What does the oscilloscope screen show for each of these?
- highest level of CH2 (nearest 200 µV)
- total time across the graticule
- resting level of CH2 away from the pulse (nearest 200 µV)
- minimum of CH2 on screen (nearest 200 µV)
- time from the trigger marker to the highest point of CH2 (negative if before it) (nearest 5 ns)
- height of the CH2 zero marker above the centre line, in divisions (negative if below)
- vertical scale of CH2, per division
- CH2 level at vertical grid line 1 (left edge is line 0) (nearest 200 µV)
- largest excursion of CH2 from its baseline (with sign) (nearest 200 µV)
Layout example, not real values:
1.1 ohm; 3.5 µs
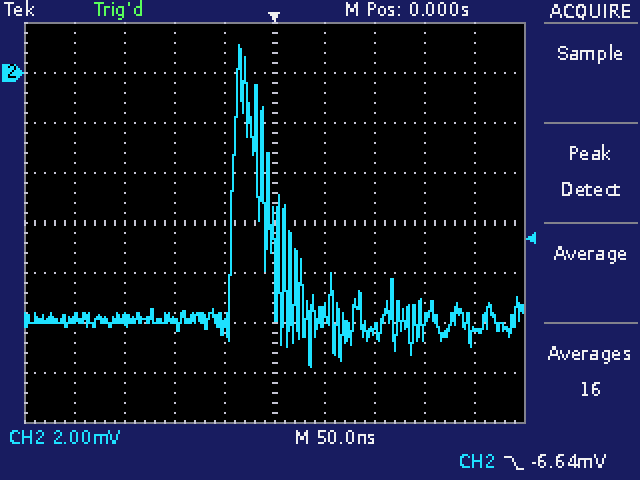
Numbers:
1.2 mV; 500 ns; -9.8 mV; -11.8 mV; -35 ns; +3.0 div; 2 mV; -9.8 mV; +11.0 mV
